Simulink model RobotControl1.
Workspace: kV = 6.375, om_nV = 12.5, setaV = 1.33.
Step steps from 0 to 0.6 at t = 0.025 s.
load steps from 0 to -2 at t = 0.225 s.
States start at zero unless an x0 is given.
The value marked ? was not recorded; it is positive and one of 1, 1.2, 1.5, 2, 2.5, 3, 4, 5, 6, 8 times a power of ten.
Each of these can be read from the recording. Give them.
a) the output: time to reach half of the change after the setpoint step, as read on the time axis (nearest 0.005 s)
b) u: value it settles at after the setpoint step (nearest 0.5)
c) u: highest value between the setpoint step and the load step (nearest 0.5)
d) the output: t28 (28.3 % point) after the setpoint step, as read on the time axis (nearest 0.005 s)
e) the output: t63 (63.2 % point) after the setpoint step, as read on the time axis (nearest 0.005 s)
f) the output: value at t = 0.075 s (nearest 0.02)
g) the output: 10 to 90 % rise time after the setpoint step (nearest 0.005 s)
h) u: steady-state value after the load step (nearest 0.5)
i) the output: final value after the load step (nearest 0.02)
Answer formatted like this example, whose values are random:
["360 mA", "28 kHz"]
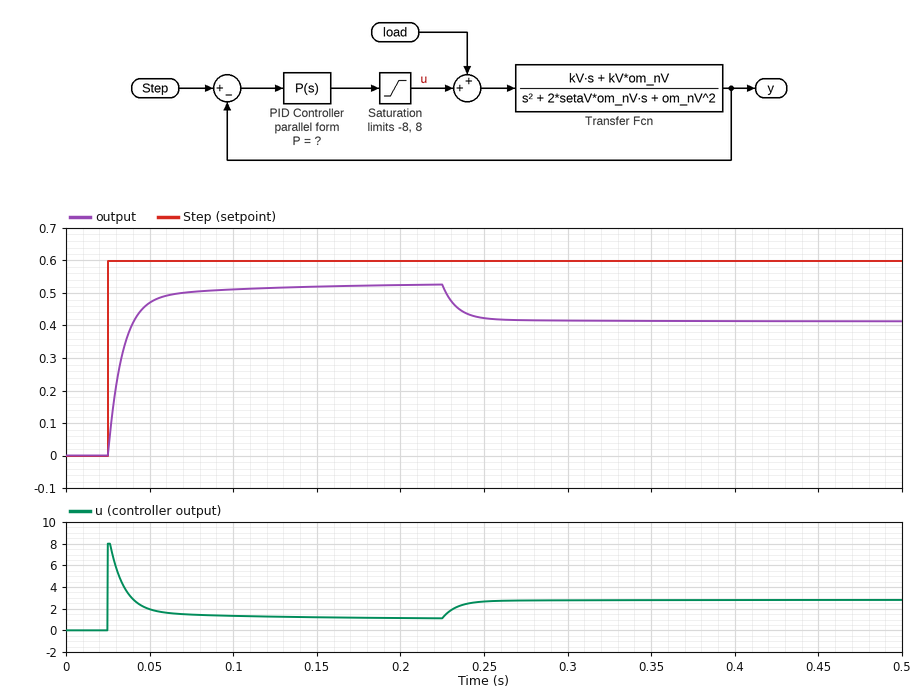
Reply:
["0.030 s", "1.0", "8.0", "0.030 s", "0.035 s", "0.50", "0.025 s", "3.0", "0.42"]
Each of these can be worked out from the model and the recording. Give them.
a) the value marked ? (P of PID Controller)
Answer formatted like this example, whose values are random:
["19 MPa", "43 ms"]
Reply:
["15"]
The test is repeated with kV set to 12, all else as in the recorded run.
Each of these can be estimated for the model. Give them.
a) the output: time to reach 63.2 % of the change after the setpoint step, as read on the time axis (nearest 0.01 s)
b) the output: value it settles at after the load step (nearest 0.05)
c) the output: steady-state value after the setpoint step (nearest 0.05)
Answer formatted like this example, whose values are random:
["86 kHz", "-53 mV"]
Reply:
["0.03 s", "0.45", "0.55"]
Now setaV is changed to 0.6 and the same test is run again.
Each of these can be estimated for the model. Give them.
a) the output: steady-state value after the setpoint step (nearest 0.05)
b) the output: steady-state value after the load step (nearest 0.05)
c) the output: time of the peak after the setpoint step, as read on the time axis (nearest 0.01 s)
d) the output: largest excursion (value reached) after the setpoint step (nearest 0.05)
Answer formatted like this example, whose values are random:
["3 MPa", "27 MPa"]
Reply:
["0.55", "0.40", "0.07 s", "0.55"]
